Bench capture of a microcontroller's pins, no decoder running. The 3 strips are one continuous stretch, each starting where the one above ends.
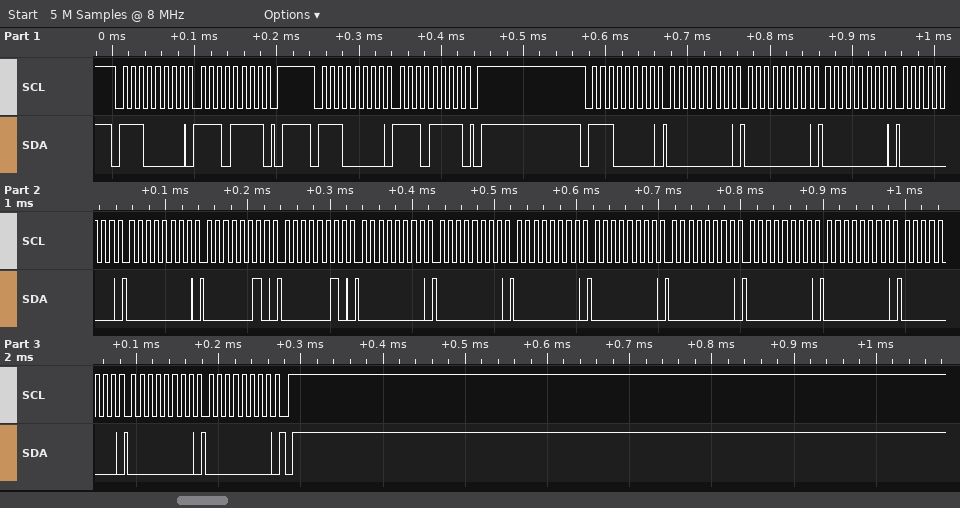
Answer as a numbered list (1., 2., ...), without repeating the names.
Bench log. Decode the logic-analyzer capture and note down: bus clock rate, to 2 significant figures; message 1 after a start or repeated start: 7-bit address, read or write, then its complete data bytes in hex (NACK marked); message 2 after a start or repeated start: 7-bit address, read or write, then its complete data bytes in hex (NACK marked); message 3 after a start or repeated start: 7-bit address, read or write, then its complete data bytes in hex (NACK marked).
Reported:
1. 100 kHz
2. 0x70 write: EF
3. 0x70 write: EF
4. 0x70 write: 00 00 00 00 00 02 02 00 00 00 00 00 00 00 00 00 00
